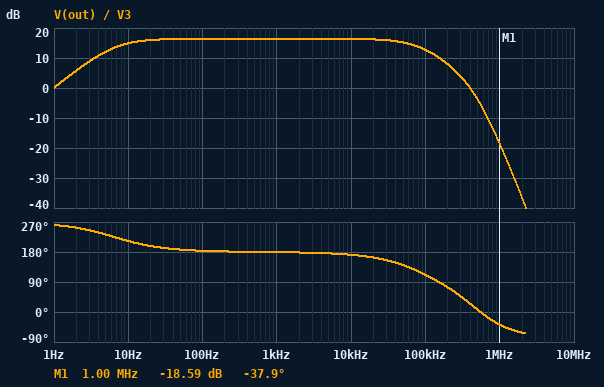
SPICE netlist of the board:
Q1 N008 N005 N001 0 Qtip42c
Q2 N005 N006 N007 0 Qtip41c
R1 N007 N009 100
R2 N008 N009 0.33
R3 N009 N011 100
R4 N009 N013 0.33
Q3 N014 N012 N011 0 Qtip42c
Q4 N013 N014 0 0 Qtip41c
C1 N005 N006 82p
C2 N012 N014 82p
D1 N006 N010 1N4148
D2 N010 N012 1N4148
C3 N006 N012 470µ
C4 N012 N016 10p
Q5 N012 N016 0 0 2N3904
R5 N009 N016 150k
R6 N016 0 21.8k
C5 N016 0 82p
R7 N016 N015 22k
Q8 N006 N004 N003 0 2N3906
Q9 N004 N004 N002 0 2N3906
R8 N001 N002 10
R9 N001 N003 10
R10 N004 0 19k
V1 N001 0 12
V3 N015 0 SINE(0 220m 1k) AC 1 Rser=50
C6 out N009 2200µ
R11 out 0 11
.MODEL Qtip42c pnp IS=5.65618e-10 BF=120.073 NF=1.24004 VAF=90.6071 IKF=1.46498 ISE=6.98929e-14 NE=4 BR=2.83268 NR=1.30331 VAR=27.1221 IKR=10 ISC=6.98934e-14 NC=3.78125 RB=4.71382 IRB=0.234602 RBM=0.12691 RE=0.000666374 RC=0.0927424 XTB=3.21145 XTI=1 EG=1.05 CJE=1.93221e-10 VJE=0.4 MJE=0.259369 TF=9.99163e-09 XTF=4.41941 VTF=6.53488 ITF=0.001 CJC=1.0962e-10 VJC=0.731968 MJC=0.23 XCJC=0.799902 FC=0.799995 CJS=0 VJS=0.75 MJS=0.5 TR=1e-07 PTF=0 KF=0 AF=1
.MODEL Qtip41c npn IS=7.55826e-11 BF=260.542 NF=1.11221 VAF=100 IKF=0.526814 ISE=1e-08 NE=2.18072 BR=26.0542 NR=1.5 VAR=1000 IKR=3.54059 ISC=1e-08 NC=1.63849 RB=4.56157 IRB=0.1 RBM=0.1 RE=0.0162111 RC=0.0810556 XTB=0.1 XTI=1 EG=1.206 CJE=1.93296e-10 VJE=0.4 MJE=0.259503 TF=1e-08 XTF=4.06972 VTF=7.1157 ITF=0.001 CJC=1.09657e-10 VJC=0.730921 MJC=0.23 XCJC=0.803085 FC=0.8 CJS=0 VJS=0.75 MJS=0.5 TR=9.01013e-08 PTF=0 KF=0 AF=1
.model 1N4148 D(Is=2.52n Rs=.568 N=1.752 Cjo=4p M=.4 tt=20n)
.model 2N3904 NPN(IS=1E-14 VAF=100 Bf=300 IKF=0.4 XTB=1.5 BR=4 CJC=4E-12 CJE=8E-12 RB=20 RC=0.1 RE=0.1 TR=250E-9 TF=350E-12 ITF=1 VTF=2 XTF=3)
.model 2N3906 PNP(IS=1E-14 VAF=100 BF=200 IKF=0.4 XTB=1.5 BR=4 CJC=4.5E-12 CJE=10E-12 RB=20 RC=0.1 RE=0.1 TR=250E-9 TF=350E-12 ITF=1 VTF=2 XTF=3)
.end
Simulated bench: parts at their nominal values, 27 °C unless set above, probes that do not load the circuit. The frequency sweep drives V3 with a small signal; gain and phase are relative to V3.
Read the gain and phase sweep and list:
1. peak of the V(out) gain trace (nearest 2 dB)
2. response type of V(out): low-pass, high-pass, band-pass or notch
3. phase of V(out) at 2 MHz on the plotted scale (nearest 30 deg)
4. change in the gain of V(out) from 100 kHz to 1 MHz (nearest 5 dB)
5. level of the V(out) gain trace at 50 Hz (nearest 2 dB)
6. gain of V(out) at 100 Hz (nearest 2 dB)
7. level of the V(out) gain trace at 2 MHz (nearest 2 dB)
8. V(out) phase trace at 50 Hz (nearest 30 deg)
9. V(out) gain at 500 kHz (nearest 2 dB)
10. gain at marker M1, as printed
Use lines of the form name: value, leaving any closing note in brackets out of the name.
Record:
peak of the V(out) gain trace: 16 dB
response type of V(out): low-pass, high-pass, band-pass or notch: band-pass
phase of V(out) at 2 MHz on the plotted scale: -60 deg
change in the gain of V(out) from 100 kHz to 1 MHz: -30 dB
level of the V(out) gain trace at 50 Hz: 16 dB
gain of V(out) at 100 Hz: 16 dB
level of the V(out) gain trace at 2 MHz: -36 dB
V(out) phase trace at 50 Hz: 180 deg
V(out) gain at 500 kHz: -4 dB
gain at marker M1, as printed: -18.59 dB
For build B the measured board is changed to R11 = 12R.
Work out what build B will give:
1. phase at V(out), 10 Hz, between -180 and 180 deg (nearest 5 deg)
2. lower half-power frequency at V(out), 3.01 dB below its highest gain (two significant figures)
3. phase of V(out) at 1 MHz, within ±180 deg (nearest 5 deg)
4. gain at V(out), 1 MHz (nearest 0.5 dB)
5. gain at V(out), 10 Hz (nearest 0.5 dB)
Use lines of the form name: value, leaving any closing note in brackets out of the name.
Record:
phase at V(out), 10 Hz, between -180 and 180 deg: -150 deg
lower half-power frequency at V(out), 3.01 dB below its highest gain: 5.9 Hz
phase of V(out) at 1 MHz, within ±180 deg: -35 deg
gain at V(out), 1 MHz: -18.0 dB
gain at V(out), 10 Hz: 15.0 dB
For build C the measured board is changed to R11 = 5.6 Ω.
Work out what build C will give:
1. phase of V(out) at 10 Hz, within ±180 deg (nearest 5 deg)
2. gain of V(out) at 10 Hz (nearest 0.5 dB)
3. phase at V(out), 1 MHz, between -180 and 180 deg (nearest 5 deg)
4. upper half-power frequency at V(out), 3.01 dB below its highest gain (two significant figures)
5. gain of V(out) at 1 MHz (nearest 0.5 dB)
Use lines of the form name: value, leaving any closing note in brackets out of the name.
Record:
phase of V(out) at 10 Hz, within ±180 deg: -130 deg
gain of V(out) at 10 Hz: 12.0 dB
phase at V(out), 1 MHz, between -180 and 180 deg: -45 deg
upper half-power frequency at V(out), 3.01 dB below its highest gain: 88 kHz
gain of V(out) at 1 MHz: -23.5 dB
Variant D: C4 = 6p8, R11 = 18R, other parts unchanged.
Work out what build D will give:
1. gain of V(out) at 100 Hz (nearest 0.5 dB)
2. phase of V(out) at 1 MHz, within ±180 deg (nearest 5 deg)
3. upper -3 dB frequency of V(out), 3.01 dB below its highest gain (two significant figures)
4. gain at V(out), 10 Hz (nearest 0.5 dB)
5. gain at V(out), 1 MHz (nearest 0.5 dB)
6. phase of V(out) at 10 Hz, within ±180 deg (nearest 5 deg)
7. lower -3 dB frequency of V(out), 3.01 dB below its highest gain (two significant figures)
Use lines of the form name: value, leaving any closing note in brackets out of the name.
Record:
gain of V(out) at 100 Hz: 16.5 dB
phase of V(out) at 1 MHz, within ±180 deg: -35 deg
upper -3 dB frequency of V(out), 3.01 dB below its highest gain: 120 kHz
gain at V(out), 10 Hz: 16.0 dB
gain at V(out), 1 MHz: -15.0 dB
phase of V(out) at 10 Hz, within ±180 deg: -160 deg
lower -3 dB frequency of V(out), 3.01 dB below its highest gain: 4.0 Hz
